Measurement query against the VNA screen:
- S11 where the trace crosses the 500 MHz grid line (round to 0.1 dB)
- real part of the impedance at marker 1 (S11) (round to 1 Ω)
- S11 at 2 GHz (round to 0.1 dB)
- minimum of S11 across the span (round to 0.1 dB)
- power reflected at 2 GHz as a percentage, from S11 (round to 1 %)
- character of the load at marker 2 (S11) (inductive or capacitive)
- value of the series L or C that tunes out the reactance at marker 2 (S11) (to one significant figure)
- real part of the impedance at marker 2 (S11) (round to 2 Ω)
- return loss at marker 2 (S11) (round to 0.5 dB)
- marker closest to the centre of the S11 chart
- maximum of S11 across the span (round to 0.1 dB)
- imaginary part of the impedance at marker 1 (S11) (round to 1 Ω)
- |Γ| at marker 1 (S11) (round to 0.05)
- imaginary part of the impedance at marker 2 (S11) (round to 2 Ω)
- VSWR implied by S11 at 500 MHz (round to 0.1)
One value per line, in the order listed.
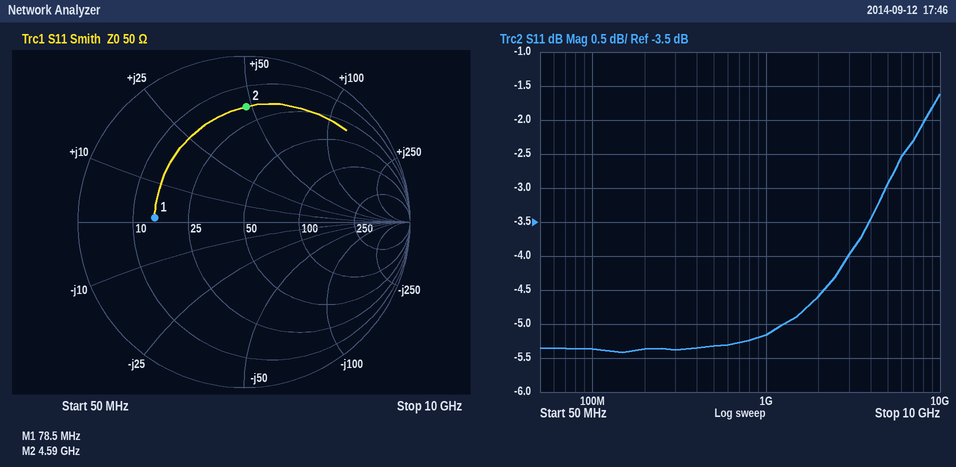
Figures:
-5.3 dB
15 Ω
-4.6 dB
-5.4 dB
35 %
inductive
700 fF
18 Ω
3.0 dB
marker 1
-1.6 dB
+1 Ω
0.55
+48 Ω
3.4
